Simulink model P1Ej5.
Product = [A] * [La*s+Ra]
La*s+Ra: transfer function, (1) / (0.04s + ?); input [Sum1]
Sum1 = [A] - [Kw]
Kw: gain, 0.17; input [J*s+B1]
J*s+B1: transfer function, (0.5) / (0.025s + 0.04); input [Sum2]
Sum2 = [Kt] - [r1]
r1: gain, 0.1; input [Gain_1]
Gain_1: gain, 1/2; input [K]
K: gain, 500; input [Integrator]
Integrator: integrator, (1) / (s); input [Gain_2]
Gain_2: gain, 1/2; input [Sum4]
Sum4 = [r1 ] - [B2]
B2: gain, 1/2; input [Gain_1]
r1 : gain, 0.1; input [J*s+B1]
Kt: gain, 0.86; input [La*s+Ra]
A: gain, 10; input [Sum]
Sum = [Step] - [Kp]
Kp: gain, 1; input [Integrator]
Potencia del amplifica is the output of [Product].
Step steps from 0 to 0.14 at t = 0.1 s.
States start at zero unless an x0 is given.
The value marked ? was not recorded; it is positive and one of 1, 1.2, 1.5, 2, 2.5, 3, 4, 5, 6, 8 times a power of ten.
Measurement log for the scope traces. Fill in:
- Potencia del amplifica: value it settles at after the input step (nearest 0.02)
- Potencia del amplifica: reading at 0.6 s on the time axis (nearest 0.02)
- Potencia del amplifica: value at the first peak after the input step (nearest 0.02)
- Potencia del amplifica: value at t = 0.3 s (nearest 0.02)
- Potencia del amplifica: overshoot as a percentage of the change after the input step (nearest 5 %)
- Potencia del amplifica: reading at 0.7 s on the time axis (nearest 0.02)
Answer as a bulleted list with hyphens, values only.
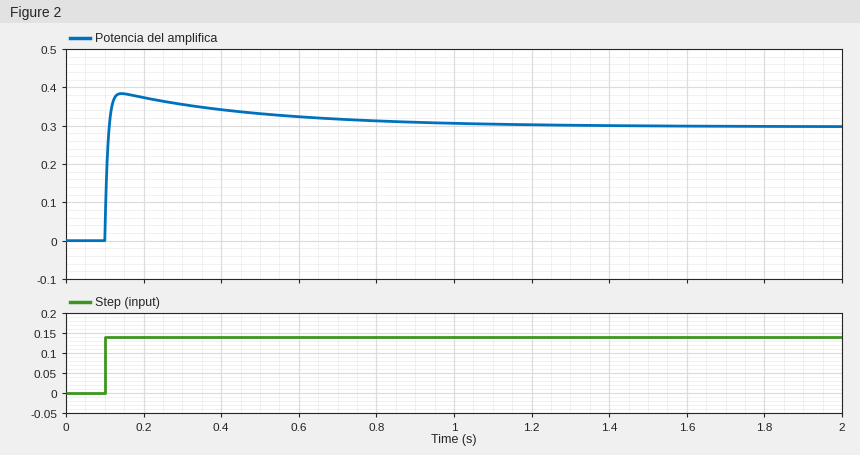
- 0.30
- 0.32
- 0.38
- 0.36
- 30 %
- 0.32
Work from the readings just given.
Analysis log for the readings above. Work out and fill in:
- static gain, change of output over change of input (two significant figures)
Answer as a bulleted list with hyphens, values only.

- 2.1
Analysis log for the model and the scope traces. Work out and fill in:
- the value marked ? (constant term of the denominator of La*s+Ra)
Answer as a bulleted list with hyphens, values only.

- 5
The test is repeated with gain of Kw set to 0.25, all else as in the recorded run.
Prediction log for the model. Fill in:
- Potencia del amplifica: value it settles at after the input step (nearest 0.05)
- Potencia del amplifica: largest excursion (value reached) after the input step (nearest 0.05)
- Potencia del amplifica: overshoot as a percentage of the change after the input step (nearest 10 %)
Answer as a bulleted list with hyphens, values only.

- 0.25
- 0.40
- 40 %
